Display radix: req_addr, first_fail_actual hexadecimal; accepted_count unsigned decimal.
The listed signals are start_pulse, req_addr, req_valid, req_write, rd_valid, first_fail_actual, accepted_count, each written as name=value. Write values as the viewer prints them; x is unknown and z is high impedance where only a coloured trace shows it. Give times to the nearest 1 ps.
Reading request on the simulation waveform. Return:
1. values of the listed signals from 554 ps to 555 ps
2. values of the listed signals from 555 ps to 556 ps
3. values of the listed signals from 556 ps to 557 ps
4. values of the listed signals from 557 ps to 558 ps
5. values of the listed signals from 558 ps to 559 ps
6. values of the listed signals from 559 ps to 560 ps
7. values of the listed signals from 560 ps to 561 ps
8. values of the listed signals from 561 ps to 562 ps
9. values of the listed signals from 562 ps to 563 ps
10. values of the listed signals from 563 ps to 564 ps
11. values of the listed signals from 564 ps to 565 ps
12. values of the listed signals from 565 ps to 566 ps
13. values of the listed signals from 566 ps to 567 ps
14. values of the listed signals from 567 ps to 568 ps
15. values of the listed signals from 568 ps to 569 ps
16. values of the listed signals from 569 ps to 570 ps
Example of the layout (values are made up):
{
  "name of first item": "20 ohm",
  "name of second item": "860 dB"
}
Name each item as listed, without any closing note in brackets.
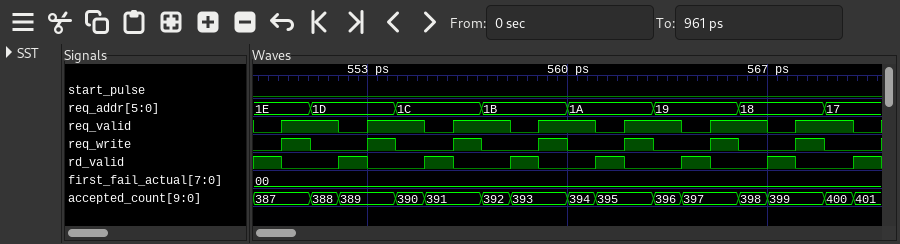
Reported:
{
  "values of the listed signals from 554 ps to 555 ps": "start_pulse=0, req_addr=1C, req_valid=1, req_write=0, rd_valid=0, first_fail_actual=00, accepted_count=390",
  "values of the listed signals from 555 ps to 556 ps": "start_pulse=0, req_addr=1C, req_valid=0, req_write=0, rd_valid=1, first_fail_actual=00, accepted_count=391",
  "values of the listed signals from 556 ps to 557 ps": "start_pulse=0, req_addr=1C, req_valid=1, req_write=1, rd_valid=0, first_fail_actual=00, accepted_count=391",
  "values of the listed signals from 557 ps to 558 ps": "start_pulse=0, req_addr=1B, req_valid=1, req_write=0, rd_valid=0, first_fail_actual=00, accepted_count=392",
  "values of the listed signals from 558 ps to 559 ps": "start_pulse=0, req_addr=1B, req_valid=0, req_write=0, rd_valid=1, first_fail_actual=00, accepted_count=393",
  "values of the listed signals from 559 ps to 560 ps": "start_pulse=0, req_addr=1B, req_valid=1, req_write=1, rd_valid=0, first_fail_actual=00, accepted_count=393",
  "values of the listed signals from 560 ps to 561 ps": "start_pulse=0, req_addr=1A, req_valid=1, req_write=0, rd_valid=0, first_fail_actual=00, accepted_count=394",
  "values of the listed signals from 561 ps to 562 ps": "start_pulse=0, req_addr=1A, req_valid=0, req_write=0, rd_valid=1, first_fail_actual=00, accepted_count=395",
  "values of the listed signals from 562 ps to 563 ps": "start_pulse=0, req_addr=1A, req_valid=1, req_write=1, rd_valid=0, first_fail_actual=00, accepted_count=395",
  "values of the listed signals from 563 ps to 564 ps": "start_pulse=0, req_addr=19, req_valid=1, req_write=0, rd_valid=0, first_fail_actual=00, accepted_count=396",
  "values of the listed signals from 564 ps to 565 ps": "start_pulse=0, req_addr=19, req_valid=0, req_write=0, rd_valid=1, first_fail_actual=00, accepted_count=397",
  "values of the listed signals from 565 ps to 566 ps": "start_pulse=0, req_addr=19, req_valid=1, req_write=1, rd_valid=0, first_fail_actual=00, accepted_count=397",
  "values of the listed signals from 566 ps to 567 ps": "start_pulse=0, req_addr=18, req_valid=1, req_write=0, rd_valid=0, first_fail_actual=00, accepted_count=398",
  "values of the listed signals from 567 ps to 568 ps": "start_pulse=0, req_addr=18, req_valid=0, req_write=0, rd_valid=1, first_fail_actual=00, accepted_count=399",
  "values of the listed signals from 568 ps to 569 ps": "start_pulse=0, req_addr=18, req_valid=1, req_write=1, rd_valid=0, first_fail_actual=00, accepted_count=399",
  "values of the listed signals from 569 ps to 570 ps": "start_pulse=0, req_addr=17, req_valid=1, req_write=0, rd_valid=0, first_fail_actual=00, accepted_count=400"
}
